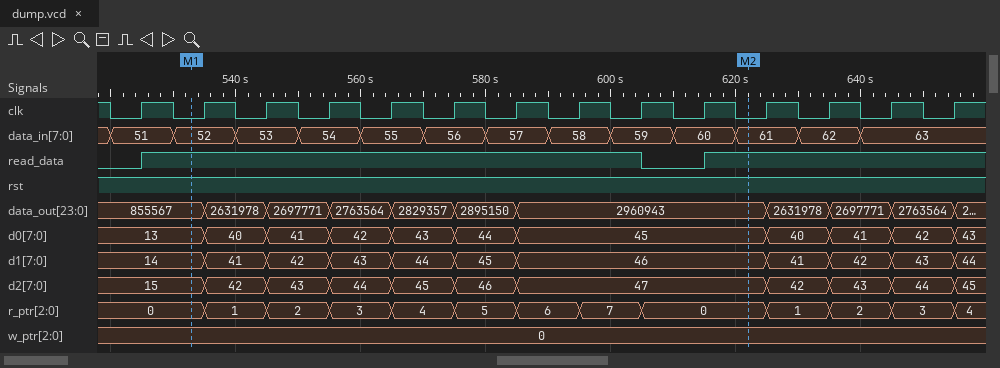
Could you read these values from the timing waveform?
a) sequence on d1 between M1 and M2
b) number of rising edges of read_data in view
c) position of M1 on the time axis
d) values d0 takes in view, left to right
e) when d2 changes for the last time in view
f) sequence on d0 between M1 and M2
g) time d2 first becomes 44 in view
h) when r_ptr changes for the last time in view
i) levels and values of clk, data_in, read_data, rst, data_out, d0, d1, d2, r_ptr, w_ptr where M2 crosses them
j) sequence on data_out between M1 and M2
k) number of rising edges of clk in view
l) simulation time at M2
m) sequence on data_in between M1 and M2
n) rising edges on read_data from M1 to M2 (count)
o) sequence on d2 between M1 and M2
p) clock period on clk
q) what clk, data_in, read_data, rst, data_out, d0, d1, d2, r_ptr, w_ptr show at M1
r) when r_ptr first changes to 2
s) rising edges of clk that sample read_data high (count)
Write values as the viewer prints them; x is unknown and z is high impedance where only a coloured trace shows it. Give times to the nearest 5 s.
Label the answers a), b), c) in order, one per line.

a) 14, 41, 42, 43, 44, 45, 46
b) 2
c) 535 s
d) 13, 40, 41, 42, 43, 44, 45, 40, 41, 42, 43
e) 655 s
f) 13, 40, 41, 42, 43, 44, 45
g) 555 s
h) 655 s
i) clk=0, data_in=61, read_data=1, rst=1, data_out=2960943, d0=45, d1=46, d2=47, r_ptr=0, w_ptr=0
j) 855567, 2631978, 2697771, 2763564, 2829357, 2895150, 2960943
k) 14
l) 620 s
m) 52, 53, 54, 55, 56, 57, 58, 59, 60, 61
n) 1
o) 15, 42, 43, 44, 45, 46, 47
p) 10 s
q) clk=0, data_in=52, read_data=1, rst=1, data_out=855567, d0=13, d1=14, d2=15, r_ptr=0, w_ptr=0
r) 545 s
s) 12
